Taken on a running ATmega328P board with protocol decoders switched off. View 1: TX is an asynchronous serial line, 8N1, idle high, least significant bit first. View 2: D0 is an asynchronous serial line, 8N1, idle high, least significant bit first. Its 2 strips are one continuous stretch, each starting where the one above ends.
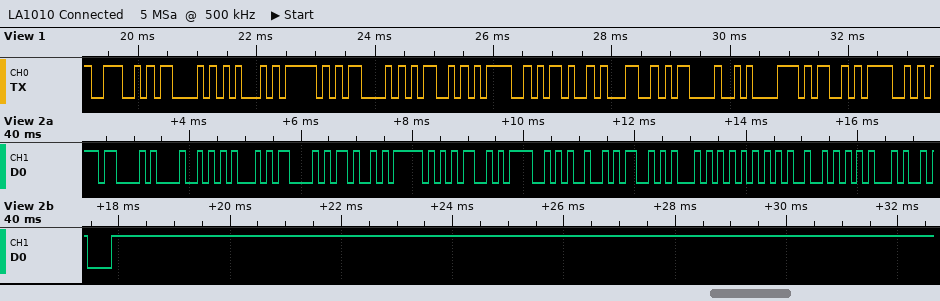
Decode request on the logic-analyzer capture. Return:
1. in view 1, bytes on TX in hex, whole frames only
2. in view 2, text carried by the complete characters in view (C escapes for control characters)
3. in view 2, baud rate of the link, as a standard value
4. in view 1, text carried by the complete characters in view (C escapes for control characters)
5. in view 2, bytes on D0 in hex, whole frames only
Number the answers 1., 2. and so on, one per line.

1. 4E 43 45 5F 43 4D 3D 2D 31 0D 0A 4D 4F
2. "CHECK_MOISTURE\n"
3. 9600 baud
4. "NCE_CM=-1\r\nMO"
5. 43 48 45 43 4B 5F 4D 4F 49 53 54 55 52 45 0A
